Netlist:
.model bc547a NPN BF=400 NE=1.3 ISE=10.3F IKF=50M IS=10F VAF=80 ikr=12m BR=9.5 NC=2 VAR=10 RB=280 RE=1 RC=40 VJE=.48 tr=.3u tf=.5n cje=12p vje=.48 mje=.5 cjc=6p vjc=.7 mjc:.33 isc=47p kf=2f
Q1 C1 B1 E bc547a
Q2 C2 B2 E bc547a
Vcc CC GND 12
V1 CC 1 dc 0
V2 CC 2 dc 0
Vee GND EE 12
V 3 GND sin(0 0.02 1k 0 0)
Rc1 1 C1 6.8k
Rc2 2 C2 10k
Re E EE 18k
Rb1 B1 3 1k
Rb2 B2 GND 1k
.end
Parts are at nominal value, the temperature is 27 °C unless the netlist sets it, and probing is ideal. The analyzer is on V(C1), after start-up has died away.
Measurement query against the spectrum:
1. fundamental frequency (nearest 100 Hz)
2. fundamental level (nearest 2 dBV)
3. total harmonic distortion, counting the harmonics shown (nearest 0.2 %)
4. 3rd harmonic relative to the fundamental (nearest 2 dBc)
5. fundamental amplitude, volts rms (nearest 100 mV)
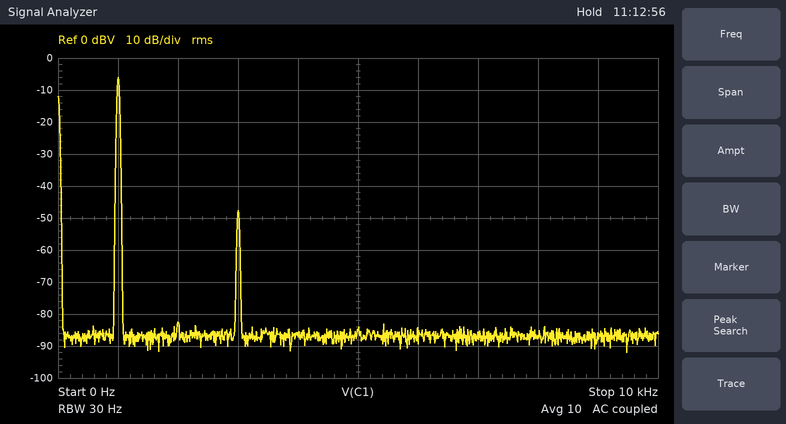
1.0 kHz
-6 dBV
0.8 %
-42 dBc
500 mV
